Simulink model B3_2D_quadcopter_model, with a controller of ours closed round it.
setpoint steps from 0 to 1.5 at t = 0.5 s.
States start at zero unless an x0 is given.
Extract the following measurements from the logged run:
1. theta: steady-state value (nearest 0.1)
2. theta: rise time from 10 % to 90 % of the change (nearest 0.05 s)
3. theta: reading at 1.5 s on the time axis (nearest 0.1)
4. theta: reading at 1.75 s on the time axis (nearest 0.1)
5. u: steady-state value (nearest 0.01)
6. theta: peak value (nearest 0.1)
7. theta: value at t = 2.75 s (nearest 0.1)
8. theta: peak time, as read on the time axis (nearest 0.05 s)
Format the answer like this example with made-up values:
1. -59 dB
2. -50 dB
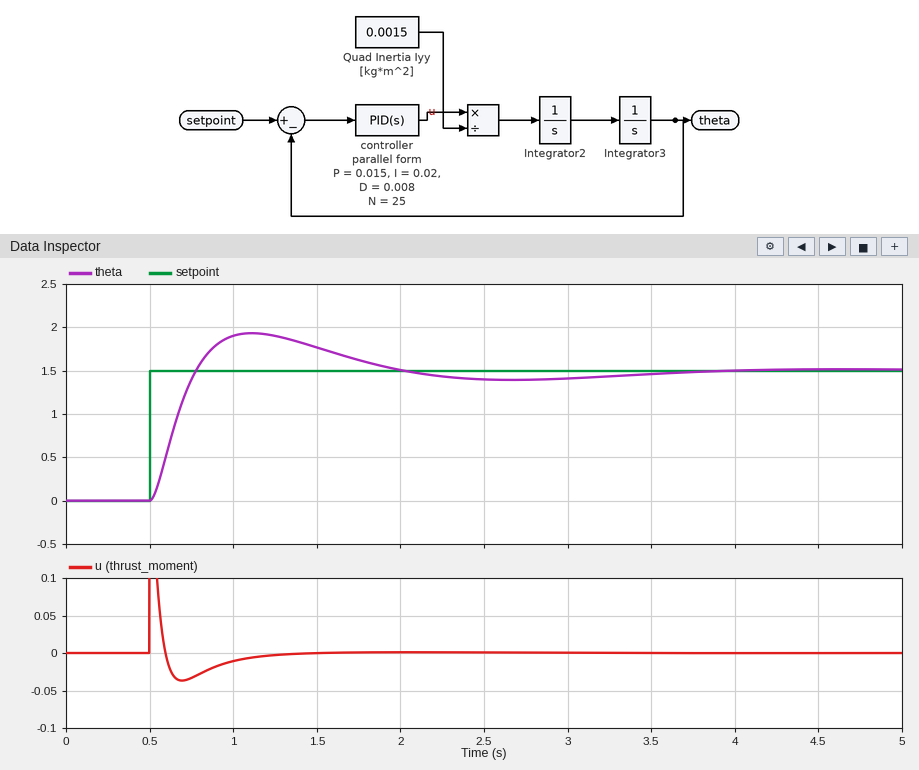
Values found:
1. 1.5
2. 0.20 s
3. 1.8
4. 1.6
5. 0.00
6. 1.9
7. 1.4
8. 1.10 s
